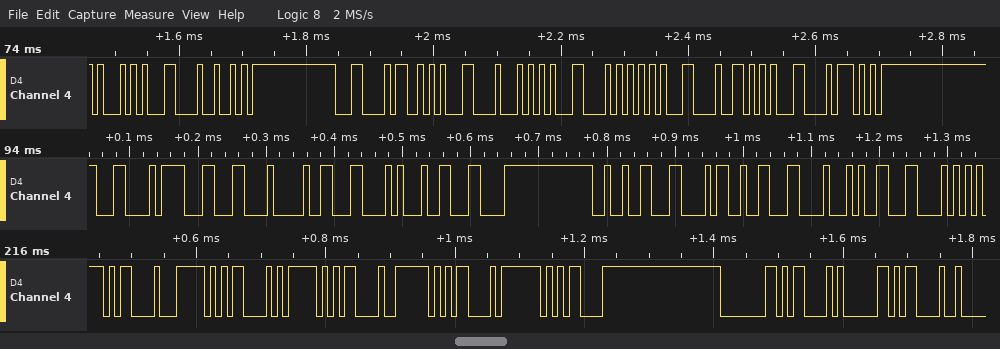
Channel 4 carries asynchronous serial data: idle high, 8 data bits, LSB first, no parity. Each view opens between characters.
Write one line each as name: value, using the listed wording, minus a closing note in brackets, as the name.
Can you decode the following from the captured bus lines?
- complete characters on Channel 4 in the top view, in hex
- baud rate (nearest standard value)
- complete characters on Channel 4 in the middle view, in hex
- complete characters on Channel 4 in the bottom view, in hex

complete characters on Channel 4 in the top view, in hex: 51, 0C, 52, 0C, 53, 0C, 54, 0C, 55, 0C, 56, 0C, 57
baud rate: 115200 baud
complete characters on Channel 4 in the middle view, in hex: 0C, 8F, 0C, 90, 0C, 91, 0C, 92, 0C, 93, 0C, 94, 0C
complete characters on Channel 4 in the bottom view, in hex: 0D, 7C, 0D, 7D, 0D, 7E, 0D, 7F, 0D, 80, 0D, 81, 0D
